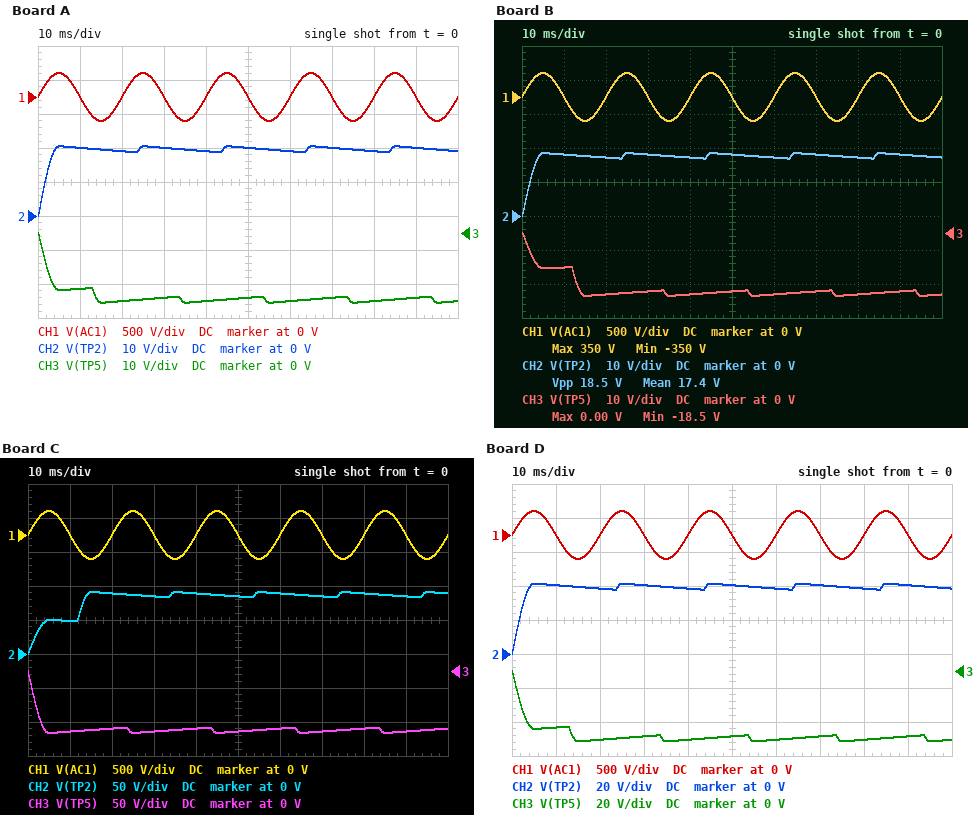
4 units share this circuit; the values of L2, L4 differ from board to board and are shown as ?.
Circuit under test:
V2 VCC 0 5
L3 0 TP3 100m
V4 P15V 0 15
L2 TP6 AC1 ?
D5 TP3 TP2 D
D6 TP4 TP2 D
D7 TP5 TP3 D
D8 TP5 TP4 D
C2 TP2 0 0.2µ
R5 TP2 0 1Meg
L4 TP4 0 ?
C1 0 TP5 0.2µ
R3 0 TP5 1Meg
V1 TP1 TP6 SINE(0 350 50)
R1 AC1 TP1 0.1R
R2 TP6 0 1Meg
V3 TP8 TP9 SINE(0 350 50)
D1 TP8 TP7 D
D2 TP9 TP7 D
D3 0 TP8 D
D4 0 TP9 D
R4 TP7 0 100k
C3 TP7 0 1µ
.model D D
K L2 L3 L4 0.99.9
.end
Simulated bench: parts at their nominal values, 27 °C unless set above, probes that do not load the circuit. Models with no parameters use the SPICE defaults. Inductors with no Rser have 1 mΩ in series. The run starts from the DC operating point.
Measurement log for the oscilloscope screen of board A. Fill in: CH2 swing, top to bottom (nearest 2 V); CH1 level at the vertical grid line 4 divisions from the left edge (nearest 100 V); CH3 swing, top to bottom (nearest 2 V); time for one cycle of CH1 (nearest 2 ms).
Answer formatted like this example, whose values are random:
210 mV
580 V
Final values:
20 V
0 V
20 V
20 ms
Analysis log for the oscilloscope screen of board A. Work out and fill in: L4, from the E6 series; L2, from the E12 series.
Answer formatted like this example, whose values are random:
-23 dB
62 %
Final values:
68 mH
27 H
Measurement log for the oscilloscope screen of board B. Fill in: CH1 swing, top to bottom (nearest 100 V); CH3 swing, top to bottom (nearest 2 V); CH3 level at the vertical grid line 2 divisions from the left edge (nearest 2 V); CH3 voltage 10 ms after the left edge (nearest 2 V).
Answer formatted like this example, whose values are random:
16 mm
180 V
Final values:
700 V
18 V
-18 V
-10 V
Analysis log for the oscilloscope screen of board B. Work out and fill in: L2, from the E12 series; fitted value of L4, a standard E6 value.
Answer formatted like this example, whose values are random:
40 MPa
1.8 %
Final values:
33 H
33 mH
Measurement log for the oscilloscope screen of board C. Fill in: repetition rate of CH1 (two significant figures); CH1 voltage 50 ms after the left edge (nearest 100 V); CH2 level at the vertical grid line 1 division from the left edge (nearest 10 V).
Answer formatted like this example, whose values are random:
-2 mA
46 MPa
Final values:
50 Hz
0 V
50 V
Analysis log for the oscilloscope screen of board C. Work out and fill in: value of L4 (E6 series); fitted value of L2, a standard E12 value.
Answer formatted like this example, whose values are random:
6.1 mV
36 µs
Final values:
330 mH
4.7 H
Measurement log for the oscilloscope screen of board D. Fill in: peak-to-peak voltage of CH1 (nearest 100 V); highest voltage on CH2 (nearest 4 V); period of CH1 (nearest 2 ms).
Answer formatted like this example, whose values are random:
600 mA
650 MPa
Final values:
700 V
40 V
20 ms
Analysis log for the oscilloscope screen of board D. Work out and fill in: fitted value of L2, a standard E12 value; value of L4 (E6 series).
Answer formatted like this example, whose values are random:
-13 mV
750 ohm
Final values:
6.8 H
68 mH
